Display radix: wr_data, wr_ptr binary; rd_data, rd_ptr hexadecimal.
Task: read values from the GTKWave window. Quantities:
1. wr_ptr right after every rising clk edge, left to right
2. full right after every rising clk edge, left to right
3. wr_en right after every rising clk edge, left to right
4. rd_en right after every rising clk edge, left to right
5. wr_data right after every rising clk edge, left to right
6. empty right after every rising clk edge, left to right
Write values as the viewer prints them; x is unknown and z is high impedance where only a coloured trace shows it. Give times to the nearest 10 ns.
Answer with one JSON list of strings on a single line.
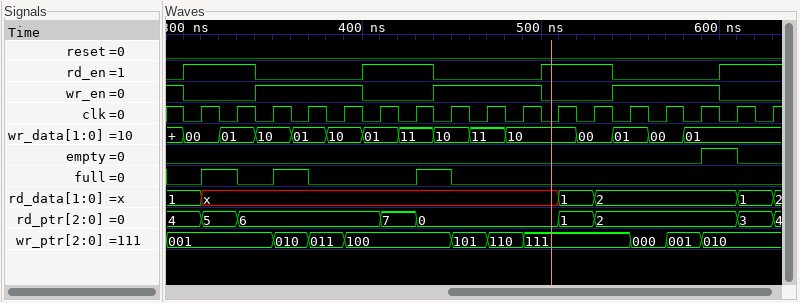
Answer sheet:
["001, 001, 010, 011, 100, 100, 100, 101, 110, 111, 111, 111, 000, 001, 010, 010, 010", "1 0 1 0 0 0 1 0 0 0 0 0 0 0 0 0 0", "0 0 1 1 1 0 0 1 1 1 0 0 1 1 1 0 0", "1 1 0 0 0 1 1 0 0 0 1 1 0 0 0 1 1", "00, 01, 10, 01, 10, 01, 11, 10, 11, 10, 10, 00, 01, 00, 01, 01, 01", "0 0 0 0 0 0 0 0 0 0 0 0 0 0 1 0 0"]
